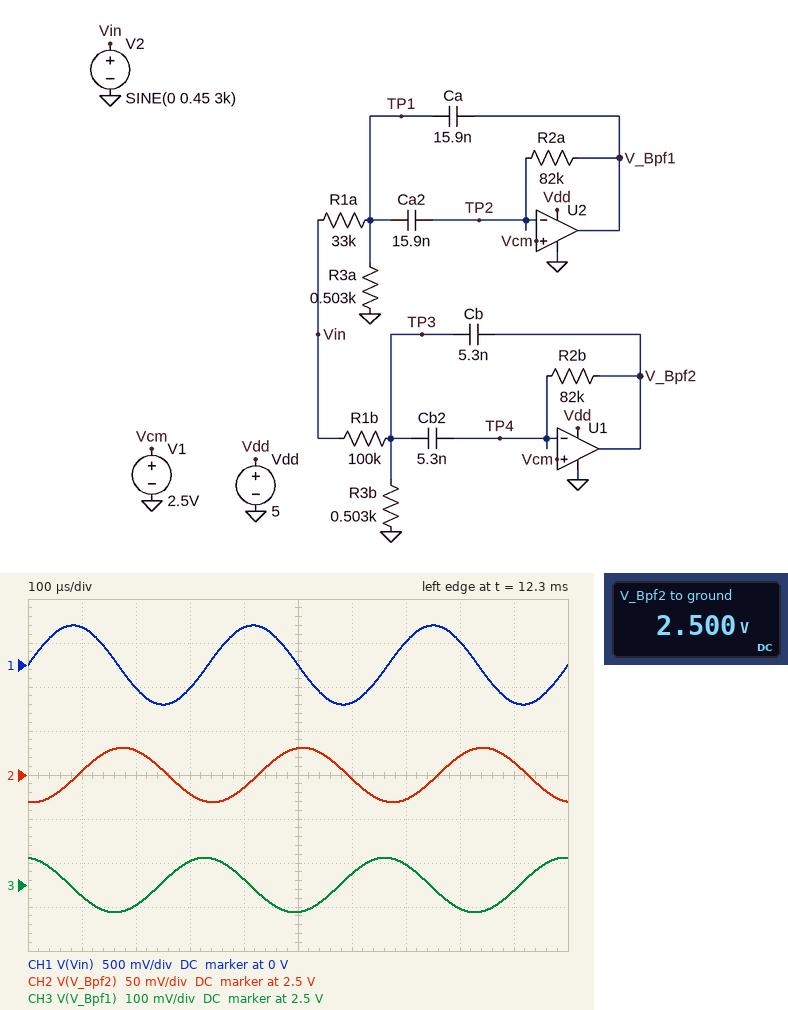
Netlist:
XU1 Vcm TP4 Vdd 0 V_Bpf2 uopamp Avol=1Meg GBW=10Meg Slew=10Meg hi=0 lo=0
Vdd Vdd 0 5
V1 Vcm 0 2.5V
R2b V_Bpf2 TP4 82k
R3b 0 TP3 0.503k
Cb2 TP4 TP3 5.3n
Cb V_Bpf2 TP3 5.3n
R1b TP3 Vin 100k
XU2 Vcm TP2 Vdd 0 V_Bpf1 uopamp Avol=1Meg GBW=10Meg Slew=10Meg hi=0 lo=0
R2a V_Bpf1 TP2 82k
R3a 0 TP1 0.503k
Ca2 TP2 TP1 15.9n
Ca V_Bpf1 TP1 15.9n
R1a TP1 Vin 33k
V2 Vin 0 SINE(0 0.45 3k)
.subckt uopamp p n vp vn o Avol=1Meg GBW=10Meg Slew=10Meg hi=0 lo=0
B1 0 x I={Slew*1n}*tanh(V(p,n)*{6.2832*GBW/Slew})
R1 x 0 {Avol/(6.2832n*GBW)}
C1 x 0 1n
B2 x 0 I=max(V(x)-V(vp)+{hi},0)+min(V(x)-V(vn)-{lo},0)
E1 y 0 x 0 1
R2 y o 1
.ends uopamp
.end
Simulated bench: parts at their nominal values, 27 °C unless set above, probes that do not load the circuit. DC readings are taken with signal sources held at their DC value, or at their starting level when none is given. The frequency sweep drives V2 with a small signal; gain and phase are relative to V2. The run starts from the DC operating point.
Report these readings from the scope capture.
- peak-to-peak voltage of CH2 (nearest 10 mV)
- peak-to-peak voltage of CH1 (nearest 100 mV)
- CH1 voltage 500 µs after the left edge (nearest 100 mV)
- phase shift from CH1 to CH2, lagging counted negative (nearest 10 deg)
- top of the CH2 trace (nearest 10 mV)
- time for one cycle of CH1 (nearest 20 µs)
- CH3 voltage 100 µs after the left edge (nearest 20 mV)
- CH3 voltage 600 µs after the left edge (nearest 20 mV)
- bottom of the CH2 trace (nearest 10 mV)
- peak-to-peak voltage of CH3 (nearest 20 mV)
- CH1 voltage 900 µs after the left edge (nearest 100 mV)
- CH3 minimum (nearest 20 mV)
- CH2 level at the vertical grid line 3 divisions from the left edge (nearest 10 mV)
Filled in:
60 mV
900 mV
0 V
-100 deg
2.53 V
340 µs
2.48 V
2.52 V
2.47 V
120 mV
-400 mV
2.44 V
2.48 V
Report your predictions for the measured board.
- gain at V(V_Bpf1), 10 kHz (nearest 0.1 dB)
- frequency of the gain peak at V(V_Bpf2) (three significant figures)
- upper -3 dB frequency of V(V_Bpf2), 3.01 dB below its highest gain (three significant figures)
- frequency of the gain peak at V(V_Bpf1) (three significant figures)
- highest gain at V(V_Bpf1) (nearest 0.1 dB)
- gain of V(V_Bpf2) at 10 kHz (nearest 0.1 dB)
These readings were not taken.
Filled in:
-30.2 dB
4.67 kHz
5.05 kHz
1.57 kHz
1.9 dB
-28.4 dB
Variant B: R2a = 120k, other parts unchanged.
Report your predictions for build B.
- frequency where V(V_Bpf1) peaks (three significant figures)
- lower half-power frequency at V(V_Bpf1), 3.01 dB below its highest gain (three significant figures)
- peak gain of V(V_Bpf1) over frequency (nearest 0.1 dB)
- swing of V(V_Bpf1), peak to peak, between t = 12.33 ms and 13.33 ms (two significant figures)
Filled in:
1.30 kHz
1.22 kHz
5.2 dB
110 mV
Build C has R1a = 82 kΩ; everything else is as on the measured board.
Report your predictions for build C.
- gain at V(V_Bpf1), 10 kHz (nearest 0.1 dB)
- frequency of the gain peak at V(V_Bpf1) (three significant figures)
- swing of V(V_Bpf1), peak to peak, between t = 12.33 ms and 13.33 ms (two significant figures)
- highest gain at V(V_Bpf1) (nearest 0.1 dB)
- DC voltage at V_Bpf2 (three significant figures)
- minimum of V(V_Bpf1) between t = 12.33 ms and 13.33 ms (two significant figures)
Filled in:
-38.1 dB
1.56 kHz
50 mV
-6.0 dB
2.50 V
2.5 V
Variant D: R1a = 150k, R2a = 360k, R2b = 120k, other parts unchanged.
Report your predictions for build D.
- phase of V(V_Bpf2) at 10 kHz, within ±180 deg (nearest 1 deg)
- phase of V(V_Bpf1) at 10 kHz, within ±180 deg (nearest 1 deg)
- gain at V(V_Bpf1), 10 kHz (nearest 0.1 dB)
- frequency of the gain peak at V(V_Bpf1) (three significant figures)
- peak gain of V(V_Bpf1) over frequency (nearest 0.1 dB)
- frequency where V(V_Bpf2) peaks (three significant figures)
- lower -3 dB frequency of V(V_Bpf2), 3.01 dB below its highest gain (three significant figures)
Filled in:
93 deg
90 deg
-43.5 dB
744 Hz
1.6 dB
3.86 kHz
3.62 kHz
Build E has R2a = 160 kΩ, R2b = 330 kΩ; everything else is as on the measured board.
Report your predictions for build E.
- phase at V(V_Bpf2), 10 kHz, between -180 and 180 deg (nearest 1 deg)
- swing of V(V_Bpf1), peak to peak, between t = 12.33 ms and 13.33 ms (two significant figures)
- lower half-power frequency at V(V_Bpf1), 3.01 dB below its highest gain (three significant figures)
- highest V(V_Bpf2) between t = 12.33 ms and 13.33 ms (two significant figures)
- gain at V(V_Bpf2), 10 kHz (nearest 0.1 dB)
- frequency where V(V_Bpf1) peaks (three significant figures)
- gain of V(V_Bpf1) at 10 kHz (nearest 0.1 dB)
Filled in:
91 deg
110 mV
1.06 kHz
2.6 V
-30.0 dB
1.12 kHz
-30.3 dB
